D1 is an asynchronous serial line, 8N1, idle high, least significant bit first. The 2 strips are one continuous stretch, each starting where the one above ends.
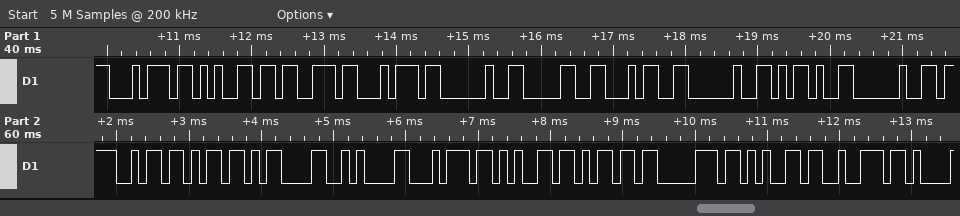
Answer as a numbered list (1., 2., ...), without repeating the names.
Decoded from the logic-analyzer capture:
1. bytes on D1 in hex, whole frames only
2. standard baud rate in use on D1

1. 74 65 73 74 20 30 34 20 2D 20 4F 6B 0D 0A 74 65 6D 70 65 72
2. 9600 baud
